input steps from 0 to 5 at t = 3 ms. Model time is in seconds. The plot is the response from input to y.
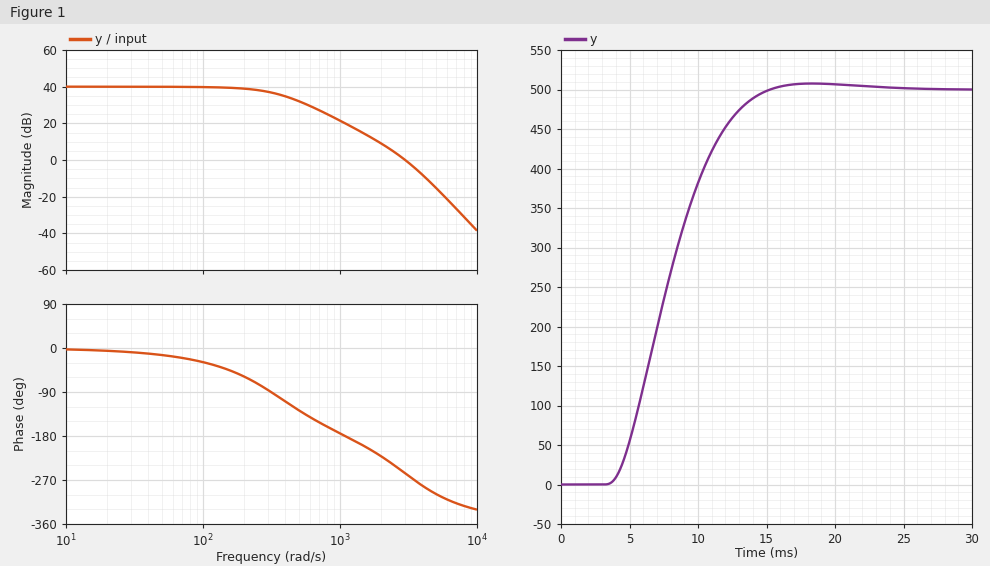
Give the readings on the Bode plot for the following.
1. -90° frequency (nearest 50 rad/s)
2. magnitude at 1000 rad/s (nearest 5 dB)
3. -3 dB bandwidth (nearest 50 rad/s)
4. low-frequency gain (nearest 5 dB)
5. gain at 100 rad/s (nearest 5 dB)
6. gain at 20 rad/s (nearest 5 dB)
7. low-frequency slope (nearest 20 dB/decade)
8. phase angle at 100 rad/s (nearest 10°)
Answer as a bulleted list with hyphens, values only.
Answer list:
- 300 rad/s
- 20 dB
- 300 rad/s
- 40 dB
- 40 dB
- 40 dB
- 0 dB/decade
- -30°
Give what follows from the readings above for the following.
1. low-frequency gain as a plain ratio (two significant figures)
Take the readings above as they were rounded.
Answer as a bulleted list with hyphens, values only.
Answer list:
- 100
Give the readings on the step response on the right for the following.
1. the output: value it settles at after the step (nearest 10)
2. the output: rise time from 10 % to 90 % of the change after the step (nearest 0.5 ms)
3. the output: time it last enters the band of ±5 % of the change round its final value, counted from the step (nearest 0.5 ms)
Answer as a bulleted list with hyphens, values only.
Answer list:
- 500
- 7.0 ms
- 10.0 ms
